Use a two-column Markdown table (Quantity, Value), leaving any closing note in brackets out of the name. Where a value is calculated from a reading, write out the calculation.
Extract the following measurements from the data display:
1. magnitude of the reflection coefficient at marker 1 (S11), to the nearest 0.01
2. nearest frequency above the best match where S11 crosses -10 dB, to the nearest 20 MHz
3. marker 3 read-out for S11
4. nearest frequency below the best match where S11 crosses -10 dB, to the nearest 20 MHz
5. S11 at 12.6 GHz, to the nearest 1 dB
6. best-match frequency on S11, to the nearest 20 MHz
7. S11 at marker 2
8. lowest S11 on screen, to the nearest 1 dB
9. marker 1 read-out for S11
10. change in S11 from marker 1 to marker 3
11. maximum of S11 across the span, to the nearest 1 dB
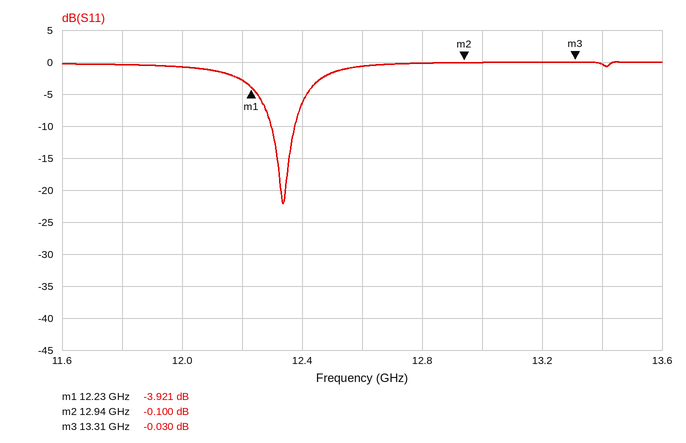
| Quantity | Value |
|---|---|
| magnitude of the reflection coefficient at marker 1 (S11), to the nearest 0.01 | 10^(-3.921/20) ≈ 0.64 |
| nearest frequency above the best match where S11 crosses -10 dB, to the nearest 20 MHz | 12.38 GHz |
| marker 3 read-out for S11 | -0.030 dB |
| nearest frequency below the best match where S11 crosses -10 dB, to the nearest 20 MHz | 12.30 GHz |
| S11 at 12.6 GHz, to the nearest 1 dB | -1 dB |
| best-match frequency on S11, to the nearest 20 MHz | 12.34 GHz |
| S11 at marker 2 | -0.100 dB |
| lowest S11 on screen, to the nearest 1 dB | -22 dB |
| marker 1 read-out for S11 | -3.921 dB |
| change in S11 from marker 1 to marker 3 | -0.03 − (-3.921) = 3.891 dB |
| maximum of S11 across the span, to the nearest 1 dB | 0 dB |
